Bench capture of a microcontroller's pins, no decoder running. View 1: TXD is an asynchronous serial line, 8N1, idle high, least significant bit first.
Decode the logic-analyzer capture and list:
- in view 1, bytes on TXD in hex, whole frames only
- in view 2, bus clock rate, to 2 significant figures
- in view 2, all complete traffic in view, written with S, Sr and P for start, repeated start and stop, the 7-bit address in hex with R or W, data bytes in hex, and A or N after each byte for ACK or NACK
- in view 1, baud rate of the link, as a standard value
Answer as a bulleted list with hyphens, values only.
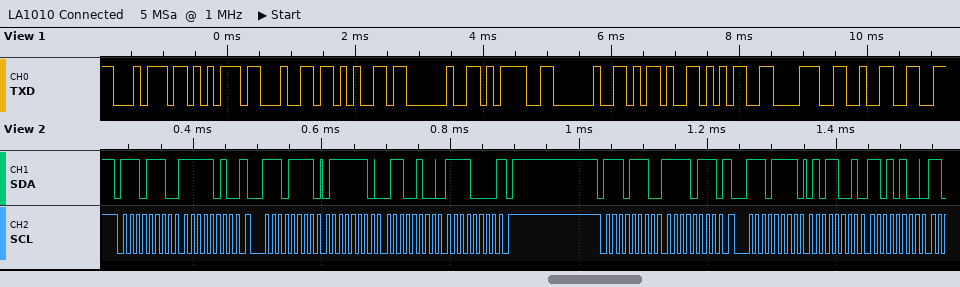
- 74 75 64 65 20 3D 20 2D 35 38 32
- 100 kHz
- S 77W A FA A Sr 77R A 7E A 64 A F0 N P S 77W A F7 A Sr 77R A 59 A D4 A
- 9600 baud
